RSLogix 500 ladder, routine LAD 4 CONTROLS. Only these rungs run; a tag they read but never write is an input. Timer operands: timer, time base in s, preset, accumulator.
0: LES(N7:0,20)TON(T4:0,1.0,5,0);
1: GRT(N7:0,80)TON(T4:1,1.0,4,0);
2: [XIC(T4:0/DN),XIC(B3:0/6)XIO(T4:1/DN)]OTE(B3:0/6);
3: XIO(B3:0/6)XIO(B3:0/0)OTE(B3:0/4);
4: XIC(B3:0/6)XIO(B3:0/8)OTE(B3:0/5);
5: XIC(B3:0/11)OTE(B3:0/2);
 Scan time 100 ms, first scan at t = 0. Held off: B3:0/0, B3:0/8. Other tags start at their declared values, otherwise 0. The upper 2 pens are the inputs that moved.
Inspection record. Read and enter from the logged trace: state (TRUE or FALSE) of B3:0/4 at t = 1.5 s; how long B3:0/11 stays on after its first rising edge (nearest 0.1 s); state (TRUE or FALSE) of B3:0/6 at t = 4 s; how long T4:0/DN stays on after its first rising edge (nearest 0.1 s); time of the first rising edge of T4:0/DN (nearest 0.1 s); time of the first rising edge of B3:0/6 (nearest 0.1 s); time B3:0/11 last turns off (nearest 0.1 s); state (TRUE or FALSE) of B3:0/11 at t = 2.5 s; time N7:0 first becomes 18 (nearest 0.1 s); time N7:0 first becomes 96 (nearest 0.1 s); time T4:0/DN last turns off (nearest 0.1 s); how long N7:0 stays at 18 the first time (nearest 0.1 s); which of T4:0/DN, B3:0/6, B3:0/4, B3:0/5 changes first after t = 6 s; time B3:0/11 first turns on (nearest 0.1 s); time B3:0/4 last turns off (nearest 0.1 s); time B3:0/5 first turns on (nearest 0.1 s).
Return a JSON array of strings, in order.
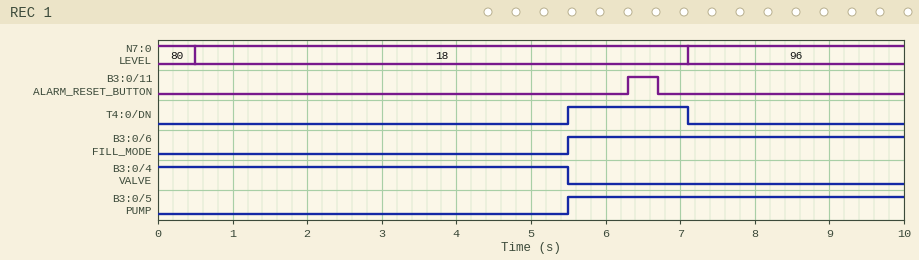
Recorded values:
["TRUE", "0.4 s", "FALSE", "1.6 s", "5.5 s", "5.5 s", "6.7 s", "FALSE", "0.5 s", "7.1 s", "7.1 s", "6.6 s", "T4:0/DN", "6.3 s", "5.5 s", "5.5 s"]
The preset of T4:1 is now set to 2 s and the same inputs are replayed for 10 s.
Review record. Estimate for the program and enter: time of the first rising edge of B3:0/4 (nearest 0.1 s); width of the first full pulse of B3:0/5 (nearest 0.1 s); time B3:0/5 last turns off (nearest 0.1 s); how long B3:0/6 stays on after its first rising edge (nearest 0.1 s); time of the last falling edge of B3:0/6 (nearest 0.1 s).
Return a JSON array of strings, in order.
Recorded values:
["9.1 s", "3.6 s", "9.1 s", "3.6 s", "9.1 s"]
